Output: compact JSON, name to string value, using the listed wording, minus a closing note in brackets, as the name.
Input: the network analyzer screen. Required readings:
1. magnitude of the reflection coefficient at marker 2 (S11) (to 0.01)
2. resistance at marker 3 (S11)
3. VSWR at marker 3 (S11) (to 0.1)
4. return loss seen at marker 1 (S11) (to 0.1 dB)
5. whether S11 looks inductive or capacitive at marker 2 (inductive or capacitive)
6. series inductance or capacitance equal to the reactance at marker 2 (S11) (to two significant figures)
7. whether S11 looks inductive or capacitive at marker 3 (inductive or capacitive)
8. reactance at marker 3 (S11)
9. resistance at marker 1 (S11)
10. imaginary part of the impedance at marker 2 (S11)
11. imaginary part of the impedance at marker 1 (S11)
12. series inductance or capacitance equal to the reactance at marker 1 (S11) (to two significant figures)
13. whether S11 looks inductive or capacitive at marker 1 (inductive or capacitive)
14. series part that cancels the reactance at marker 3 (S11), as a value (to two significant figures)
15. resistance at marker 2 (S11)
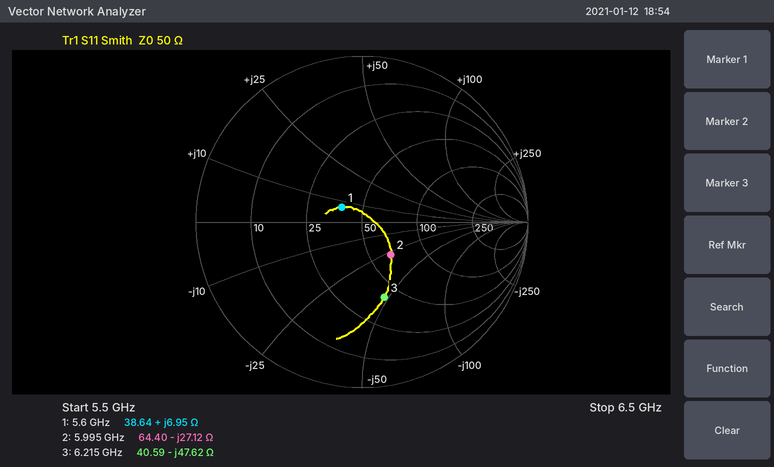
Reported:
{"magnitude of the reflection coefficient at marker 2 (S11)": "0.26", "resistance at marker 3": "40.59 Ω", "VSWR at marker 3 (S11)": "2.8", "return loss seen at marker 1 (S11)": "16.5 dB", "whether S11 looks inductive or capacitive at marker 2": "capacitive", "series inductance or capacitance equal to the reactance at marker 2 (S11)": "980 fF", "whether S11 looks inductive or capacitive at marker 3": "capacitive", "reactance at marker 3": "-47.62 Ω", "resistance at marker 1": "38.64 Ω", "imaginary part of the impedance at marker 2": "-27.12 Ω", "imaginary part of the impedance at marker 1": "+6.95 Ω", "series inductance or capacitance equal to the reactance at marker 1 (S11)": "200 pH", "whether S11 looks inductive or capacitive at marker 1": "inductive", "series part that cancels the reactance at marker 3 (S11), as a value": "1.2 nH", "resistance at marker 2": "64.40 Ω"}
